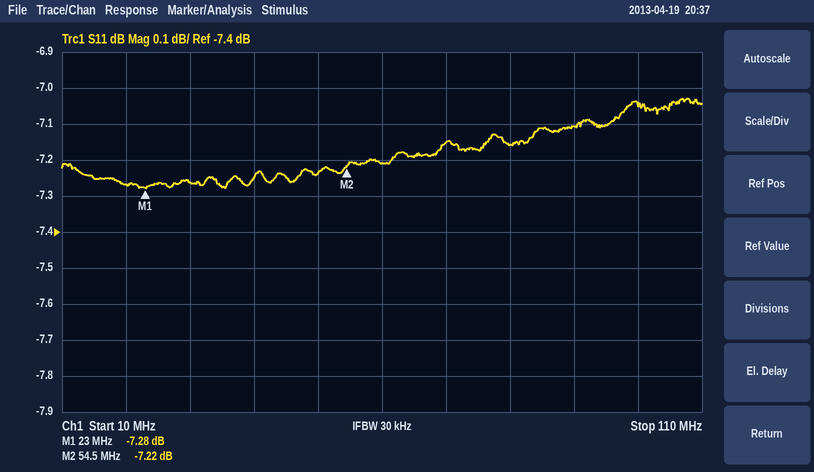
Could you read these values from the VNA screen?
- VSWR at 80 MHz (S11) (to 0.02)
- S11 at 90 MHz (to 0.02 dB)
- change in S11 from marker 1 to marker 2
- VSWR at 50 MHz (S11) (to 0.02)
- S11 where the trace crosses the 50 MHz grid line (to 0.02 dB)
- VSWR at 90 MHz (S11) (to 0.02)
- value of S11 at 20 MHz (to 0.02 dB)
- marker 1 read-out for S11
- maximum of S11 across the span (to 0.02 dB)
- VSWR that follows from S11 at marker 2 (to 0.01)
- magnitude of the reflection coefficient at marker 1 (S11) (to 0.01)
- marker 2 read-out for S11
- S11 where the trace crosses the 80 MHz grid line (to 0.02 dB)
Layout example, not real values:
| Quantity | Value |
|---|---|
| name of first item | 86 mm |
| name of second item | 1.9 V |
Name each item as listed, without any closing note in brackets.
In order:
| Quantity | Value |
|---|---|
| VSWR at 80 MHz (S11) | 2.56 |
| S11 at 90 MHz | -7.10 dB |
| change in S11 from marker 1 to marker 2 | 0.06 dB |
| VSWR at 50 MHz (S11) | 2.54 |
| S11 where the trace crosses the 50 MHz grid line | -7.24 dB |
| VSWR at 90 MHz (S11) | 2.58 |
| value of S11 at 20 MHz | -7.26 dB |
| marker 1 read-out for S11 | -7.28 dB |
| maximum of S11 across the span | -7.02 dB |
| VSWR that follows from S11 at marker 2 | 2.54 |
| magnitude of the reflection coefficient at marker 1 (S11) | 0.43 |
| marker 2 read-out for S11 | -7.22 dB |
| S11 where the trace crosses the 80 MHz grid line | -7.16 dB |
